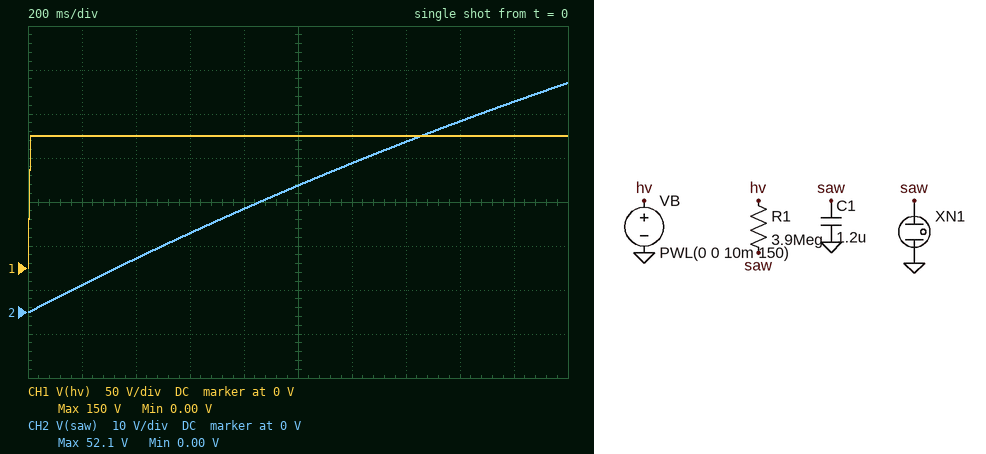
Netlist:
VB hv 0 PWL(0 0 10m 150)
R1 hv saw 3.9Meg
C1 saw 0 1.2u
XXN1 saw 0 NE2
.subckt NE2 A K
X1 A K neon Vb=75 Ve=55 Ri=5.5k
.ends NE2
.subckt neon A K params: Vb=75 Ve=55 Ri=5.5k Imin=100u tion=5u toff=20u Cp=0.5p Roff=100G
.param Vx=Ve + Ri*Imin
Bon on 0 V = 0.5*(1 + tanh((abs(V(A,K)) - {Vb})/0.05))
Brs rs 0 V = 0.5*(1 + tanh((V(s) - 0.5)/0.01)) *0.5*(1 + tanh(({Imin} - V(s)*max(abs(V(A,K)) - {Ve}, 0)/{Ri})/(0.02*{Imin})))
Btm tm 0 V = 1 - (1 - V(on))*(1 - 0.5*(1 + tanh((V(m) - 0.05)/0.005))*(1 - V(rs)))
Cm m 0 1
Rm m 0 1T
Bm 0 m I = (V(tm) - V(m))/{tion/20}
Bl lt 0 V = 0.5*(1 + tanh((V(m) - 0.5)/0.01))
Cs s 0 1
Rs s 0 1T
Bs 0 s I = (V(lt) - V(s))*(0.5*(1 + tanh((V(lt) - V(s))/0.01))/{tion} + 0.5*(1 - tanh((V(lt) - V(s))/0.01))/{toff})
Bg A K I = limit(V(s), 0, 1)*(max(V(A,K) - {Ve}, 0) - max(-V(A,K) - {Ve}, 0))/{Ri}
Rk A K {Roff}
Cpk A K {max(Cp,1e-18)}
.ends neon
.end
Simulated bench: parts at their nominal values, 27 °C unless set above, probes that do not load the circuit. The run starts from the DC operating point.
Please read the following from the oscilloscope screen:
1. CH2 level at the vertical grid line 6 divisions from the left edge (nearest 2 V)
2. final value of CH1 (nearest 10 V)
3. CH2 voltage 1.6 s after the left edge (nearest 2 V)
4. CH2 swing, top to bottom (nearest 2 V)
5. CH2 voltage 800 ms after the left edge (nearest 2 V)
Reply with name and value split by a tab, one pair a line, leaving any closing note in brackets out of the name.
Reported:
CH2 level at the vertical grid line 6 divisions from the left edge	34 V
final value of CH1	150 V
CH2 voltage 1.6 s after the left edge	44 V
CH2 swing, top to bottom	52 V
CH2 voltage 800 ms after the left edge	24 V
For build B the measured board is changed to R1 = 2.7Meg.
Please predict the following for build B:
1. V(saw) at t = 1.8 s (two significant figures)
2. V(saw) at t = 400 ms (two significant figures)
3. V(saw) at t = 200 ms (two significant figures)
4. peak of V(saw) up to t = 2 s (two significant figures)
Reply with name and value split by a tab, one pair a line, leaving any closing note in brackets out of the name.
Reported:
V(saw) at t = 1.8 s	64 V
V(saw) at t = 400 ms	17 V
V(saw) at t = 200 ms	8.8 V
peak of V(saw) up to t = 2 s	69 V
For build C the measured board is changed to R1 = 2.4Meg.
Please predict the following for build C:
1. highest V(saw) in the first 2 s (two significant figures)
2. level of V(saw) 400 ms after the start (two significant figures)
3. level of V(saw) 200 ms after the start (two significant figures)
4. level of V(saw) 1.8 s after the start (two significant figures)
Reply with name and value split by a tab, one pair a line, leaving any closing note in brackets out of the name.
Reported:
highest V(saw) in the first 2 s	75 V
level of V(saw) 400 ms after the start	19 V
level of V(saw) 200 ms after the start	9.8 V
level of V(saw) 1.8 s after the start	70 V
